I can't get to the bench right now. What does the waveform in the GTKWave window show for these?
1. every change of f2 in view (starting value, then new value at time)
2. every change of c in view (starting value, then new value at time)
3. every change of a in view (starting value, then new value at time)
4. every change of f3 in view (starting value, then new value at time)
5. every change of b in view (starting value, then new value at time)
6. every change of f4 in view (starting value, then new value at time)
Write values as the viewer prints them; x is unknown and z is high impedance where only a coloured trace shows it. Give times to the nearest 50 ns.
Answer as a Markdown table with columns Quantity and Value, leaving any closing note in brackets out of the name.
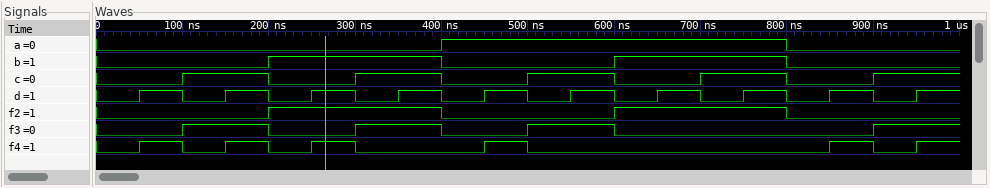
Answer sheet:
| Quantity | Value |
|---|---|
| every change of f2 in view | 0, 1 at 200 ns, 0 at 400 ns, 1 at 600 ns, 0 at 800 ns |
| every change of c in view | 0, 1 at 100 ns, 0 at 200 ns, 1 at 300 ns, 0 at 400 ns, 1 at 500 ns, 0 at 600 ns, 1 at 700 ns, 0 at 800 ns, 1 at 900 ns |
| every change of a in view | 0, 1 at 400 ns, 0 at 800 ns |
| every change of f3 in view | 0, 1 at 100 ns, 0 at 200 ns, 1 at 300 ns, 0 at 400 ns, 1 at 500 ns, 0 at 600 ns, 1 at 900 ns |
| every change of b in view | 0, 1 at 200 ns, 0 at 400 ns, 1 at 600 ns, 0 at 800 ns |
| every change of f4 in view | 0, 1 at 50 ns, 0 at 100 ns, 1 at 150 ns, 0 at 200 ns, 1 at 250 ns, 0 at 300 ns, 1 at 450 ns, 0 at 500 ns, 1 at 850 ns, 0 at 900 ns, 1 at 950 ns |
